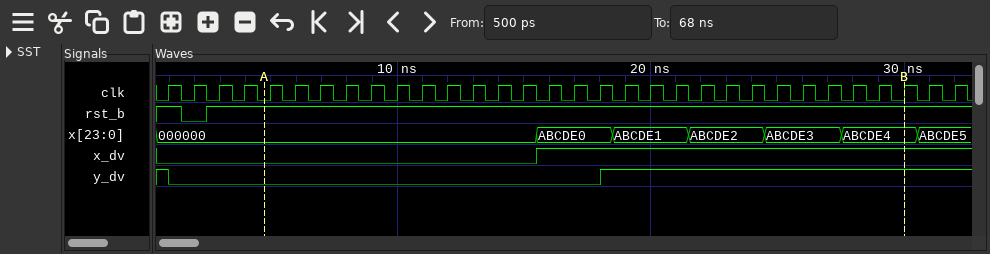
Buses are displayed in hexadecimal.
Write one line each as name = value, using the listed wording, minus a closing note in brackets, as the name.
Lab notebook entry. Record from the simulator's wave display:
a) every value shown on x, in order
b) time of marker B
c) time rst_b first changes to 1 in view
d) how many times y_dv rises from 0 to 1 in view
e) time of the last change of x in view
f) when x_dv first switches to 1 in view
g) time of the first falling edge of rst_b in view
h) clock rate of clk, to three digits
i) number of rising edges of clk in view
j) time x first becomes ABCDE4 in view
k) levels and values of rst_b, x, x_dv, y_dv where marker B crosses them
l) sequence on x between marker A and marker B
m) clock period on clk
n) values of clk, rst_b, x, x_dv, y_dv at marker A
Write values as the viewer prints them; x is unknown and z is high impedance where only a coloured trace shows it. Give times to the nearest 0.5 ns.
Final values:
every value shown on x, in order = 000000, ABCDE0, ABCDE1, ABCDE2, ABCDE3, ABCDE4, ABCDE5
time of marker B = 30 ns
time rst_b first changes to 1 in view = 2.5 ns
how many times y_dv rises from 0 to 1 in view = 1
time of the last change of x in view = 30.5 ns
when x_dv first switches to 1 in view = 15.5 ns
time of the first falling edge of rst_b in view = 1.5 ns
clock rate of clk, to three digits = 1.00 GHz
number of rising edges of clk in view = 32
time x first becomes ABCDE4 in view = 27.5 ns
levels and values of rst_b, x, x_dv, y_dv where marker B crosses them = rst_b=1, x=ABCDE4, x_dv=1, y_dv=1
sequence on x between marker A and marker B = 000000, ABCDE0, ABCDE1, ABCDE2, ABCDE3, ABCDE4
clock period on clk = 1 ns
values of clk, rst_b, x, x_dv, y_dv at marker A = clk=0, rst_b=1, x=000000, x_dv=0, y_dv=0
